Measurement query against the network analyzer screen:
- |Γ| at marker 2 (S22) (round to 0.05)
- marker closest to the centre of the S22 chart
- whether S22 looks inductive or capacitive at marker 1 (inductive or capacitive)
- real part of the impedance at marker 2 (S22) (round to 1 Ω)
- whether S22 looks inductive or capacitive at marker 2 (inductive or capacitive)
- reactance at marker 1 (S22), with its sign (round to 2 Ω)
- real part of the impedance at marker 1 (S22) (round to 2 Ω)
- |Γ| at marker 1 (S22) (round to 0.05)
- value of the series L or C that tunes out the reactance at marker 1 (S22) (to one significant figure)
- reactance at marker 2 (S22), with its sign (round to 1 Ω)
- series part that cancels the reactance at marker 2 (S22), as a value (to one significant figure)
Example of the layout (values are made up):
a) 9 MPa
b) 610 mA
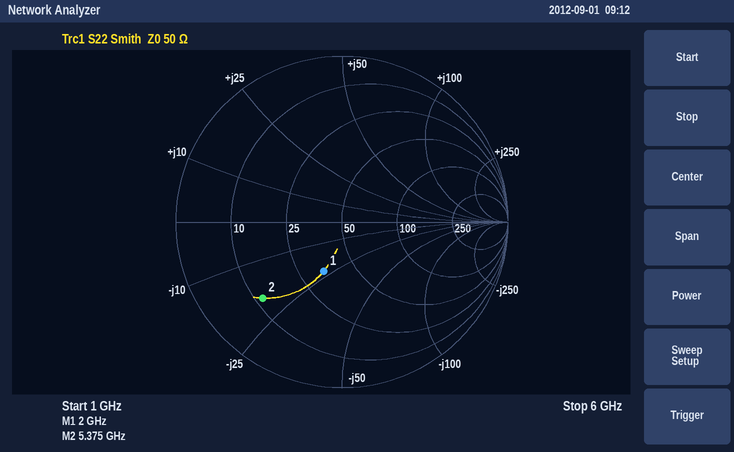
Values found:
a) 0.65
b) marker 1
c) capacitive
d) 12 Ω
e) capacitive
f) -22 Ω
g) 34 Ω
h) 0.30
i) 2 nH
j) -19 Ω
k) 600 pH
